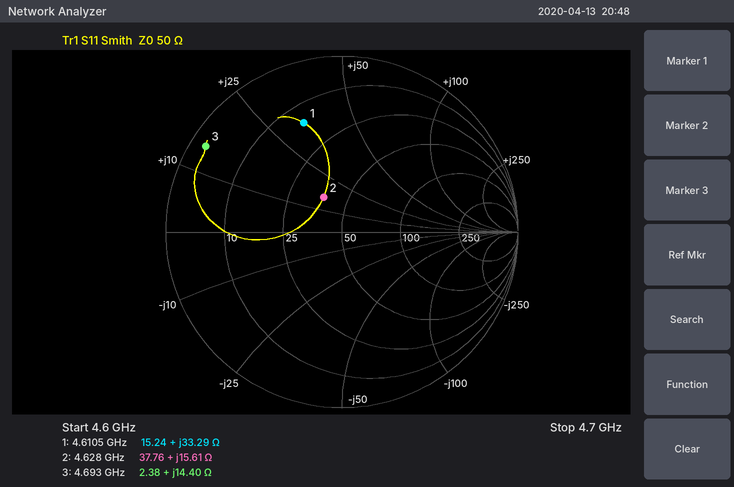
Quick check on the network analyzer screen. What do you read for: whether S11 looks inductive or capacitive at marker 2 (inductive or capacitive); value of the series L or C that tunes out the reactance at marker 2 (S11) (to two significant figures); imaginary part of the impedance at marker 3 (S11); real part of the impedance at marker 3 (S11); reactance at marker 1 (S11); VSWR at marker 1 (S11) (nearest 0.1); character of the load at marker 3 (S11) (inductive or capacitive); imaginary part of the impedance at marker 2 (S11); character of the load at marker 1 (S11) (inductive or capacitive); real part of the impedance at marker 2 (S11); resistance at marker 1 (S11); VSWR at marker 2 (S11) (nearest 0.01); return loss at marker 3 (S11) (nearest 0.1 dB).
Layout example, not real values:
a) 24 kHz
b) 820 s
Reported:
a) inductive
b) 2.2 pF
c) +14.40 Ω
d) 2.38 Ω
e) +33.29 Ω
f) 4.8
g) inductive
h) +15.61 Ω
i) inductive
j) 37.76 Ω
k) 15.24 Ω
l) 1.57
m) 0.8 dB
